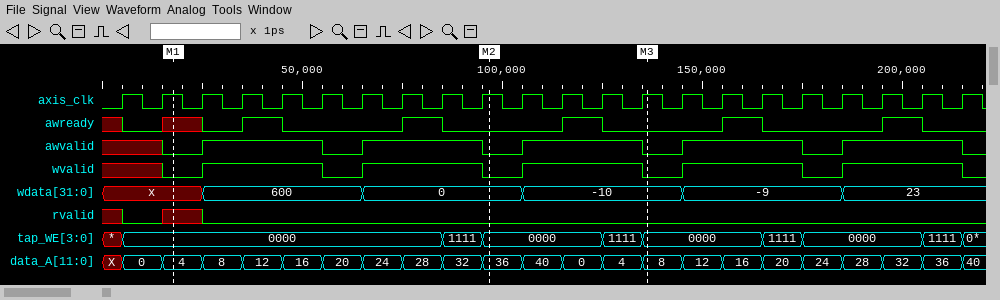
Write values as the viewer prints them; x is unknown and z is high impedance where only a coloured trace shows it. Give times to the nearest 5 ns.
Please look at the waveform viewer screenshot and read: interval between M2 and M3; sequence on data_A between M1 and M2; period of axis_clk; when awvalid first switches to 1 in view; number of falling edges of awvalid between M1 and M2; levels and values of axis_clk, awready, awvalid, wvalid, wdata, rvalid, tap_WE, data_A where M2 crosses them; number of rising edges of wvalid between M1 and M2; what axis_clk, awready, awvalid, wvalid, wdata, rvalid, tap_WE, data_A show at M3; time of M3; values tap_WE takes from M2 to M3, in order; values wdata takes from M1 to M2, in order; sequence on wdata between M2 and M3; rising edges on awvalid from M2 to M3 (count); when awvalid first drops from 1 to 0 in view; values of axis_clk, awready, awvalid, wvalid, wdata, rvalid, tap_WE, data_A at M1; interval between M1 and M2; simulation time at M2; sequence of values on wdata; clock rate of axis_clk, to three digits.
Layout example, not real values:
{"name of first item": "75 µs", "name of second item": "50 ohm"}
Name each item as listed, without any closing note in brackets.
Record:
{"interval between M2 and M3": "40 ns", "sequence on data_A between M1 and M2": "4, 8, 12, 16, 20, 24, 28, 32, 36", "period of axis_clk": "10 ns", "when awvalid first switches to 1 in view": "25 ns", "number of falling edges of awvalid between M1 and M2": "2", "levels and values of axis_clk, awready, awvalid, wvalid, wdata, rvalid, tap_WE, data_A where M2 crosses them": "axis_clk=1, awready=0, awvalid=0, wvalid=0, wdata=0, rvalid=0, tap_WE=0000, data_A=36", "number of rising edges of wvalid between M1 and M2": "2", "what axis_clk, awready, awvalid, wvalid, wdata, rvalid, tap_WE, data_A show at M3": "axis_clk=1, awready=0, awvalid=0, wvalid=0, wdata=-10, rvalid=0, tap_WE=0000, data_A=8", "time of M3": "135 ns", "values tap_WE takes from M2 to M3, in order": "0000, 1111, 0000", "values wdata takes from M1 to M2, in order": "x, 600, 0", "sequence on wdata between M2 and M3": "0, -10", "rising edges on awvalid from M2 to M3": "1", "when awvalid first drops from 1 to 0 in view": "55 ns", "values of axis_clk, awready, awvalid, wvalid, wdata, rvalid, tap_WE, data_A at M1": "axis_clk=1, awready=x, awvalid=0, wvalid=0, wdata=x, rvalid=x, tap_WE=0000, data_A=4", "interval between M1 and M2": "80 ns", "simulation time at M2": "95 ns", "sequence of values on wdata": "x, 600, 0, -10, -9, 23", "clock rate of axis_clk, to three digits": "100 MHz"}
